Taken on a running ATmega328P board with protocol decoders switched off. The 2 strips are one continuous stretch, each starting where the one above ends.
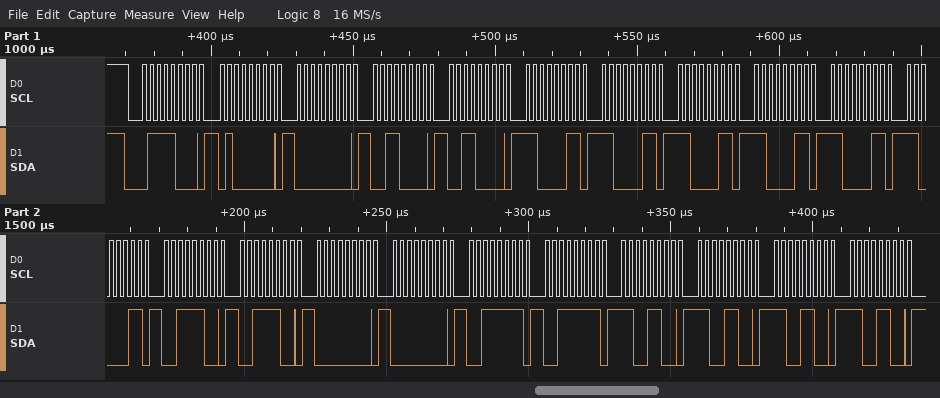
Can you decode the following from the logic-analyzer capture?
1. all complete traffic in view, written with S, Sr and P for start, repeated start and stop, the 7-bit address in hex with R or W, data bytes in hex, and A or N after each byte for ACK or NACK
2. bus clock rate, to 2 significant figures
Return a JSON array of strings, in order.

["S 3CW A 40 A 00 A 30 A 30 A C3 A C3 A C3 A C3 A C3 A C3 A 3C A 3C A 00 A 00 A 3F A 3F A CC A CC A CC A CC A", "400 kHz"]
